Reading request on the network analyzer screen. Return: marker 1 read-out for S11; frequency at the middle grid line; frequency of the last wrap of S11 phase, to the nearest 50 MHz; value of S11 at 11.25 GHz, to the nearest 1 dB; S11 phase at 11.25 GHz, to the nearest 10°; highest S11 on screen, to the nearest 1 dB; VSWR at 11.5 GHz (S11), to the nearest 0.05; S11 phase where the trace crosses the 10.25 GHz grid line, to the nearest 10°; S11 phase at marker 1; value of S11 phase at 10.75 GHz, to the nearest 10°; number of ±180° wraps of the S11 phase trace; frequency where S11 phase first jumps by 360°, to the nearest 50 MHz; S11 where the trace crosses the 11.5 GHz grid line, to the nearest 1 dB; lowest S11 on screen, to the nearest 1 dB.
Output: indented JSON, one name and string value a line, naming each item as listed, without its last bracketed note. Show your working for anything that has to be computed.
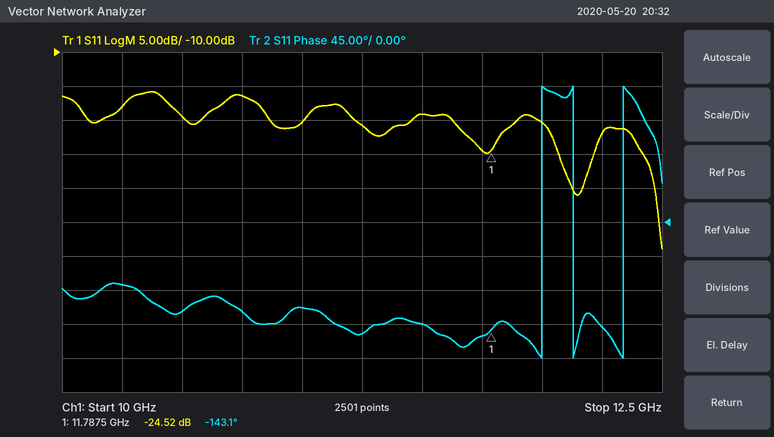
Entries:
{
  "marker 1 read-out for S11": "-24.52 dB",
  "frequency at the middle grid line": "11.25 GHz",
  "frequency of the last wrap of S11 phase, to the nearest 50 MHz": "12.35 GHz",
  "value of S11 at 11.25 GHz, to the nearest 1 dB": "-21 dB",
  "S11 phase at 11.25 GHz, to the nearest 10°": "-150°",
  "highest S11 on screen, to the nearest 1 dB": "-16 dB",
  "VSWR at 11.5 GHz (S11), to the nearest 0.05": "|Γ| = 10^(-19/20) = 0.1122; VSWR = (1 + 0.1122)/(1 − 0.1122) ≈ 1.25",
  "S11 phase where the trace crosses the 10.25 GHz grid line, to the nearest 10°": "-80°",
  "S11 phase at marker 1": "-143.1°",
  "value of S11 phase at 10.75 GHz, to the nearest 10°": "-120°",
  "number of ±180° wraps of the S11 phase trace": "3",
  "frequency where S11 phase first jumps by 360°, to the nearest 50 MHz": "12.00 GHz",
  "S11 where the trace crosses the 11.5 GHz grid line, to the nearest 1 dB": "-19 dB",
  "lowest S11 on screen, to the nearest 1 dB": "-39 dB"
}
